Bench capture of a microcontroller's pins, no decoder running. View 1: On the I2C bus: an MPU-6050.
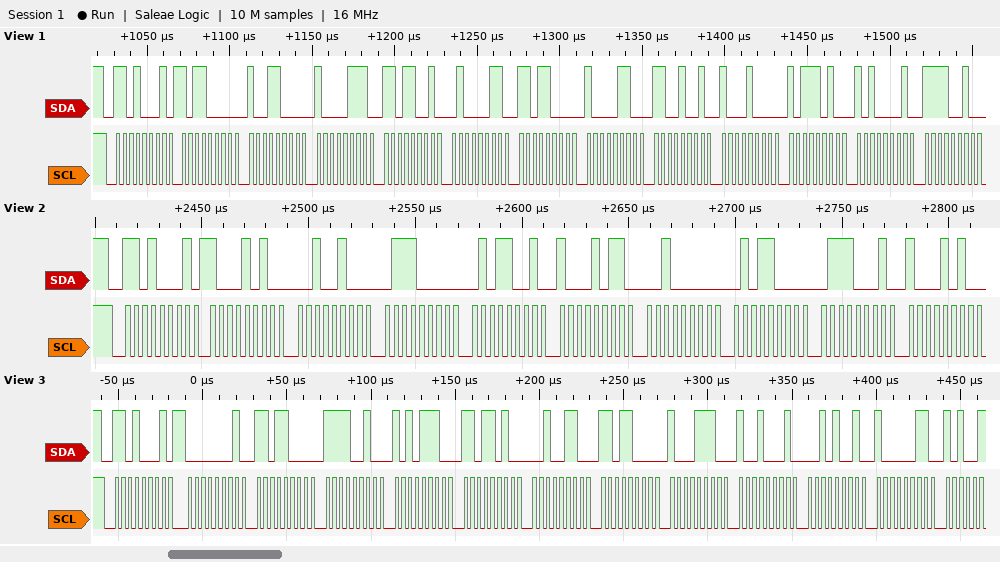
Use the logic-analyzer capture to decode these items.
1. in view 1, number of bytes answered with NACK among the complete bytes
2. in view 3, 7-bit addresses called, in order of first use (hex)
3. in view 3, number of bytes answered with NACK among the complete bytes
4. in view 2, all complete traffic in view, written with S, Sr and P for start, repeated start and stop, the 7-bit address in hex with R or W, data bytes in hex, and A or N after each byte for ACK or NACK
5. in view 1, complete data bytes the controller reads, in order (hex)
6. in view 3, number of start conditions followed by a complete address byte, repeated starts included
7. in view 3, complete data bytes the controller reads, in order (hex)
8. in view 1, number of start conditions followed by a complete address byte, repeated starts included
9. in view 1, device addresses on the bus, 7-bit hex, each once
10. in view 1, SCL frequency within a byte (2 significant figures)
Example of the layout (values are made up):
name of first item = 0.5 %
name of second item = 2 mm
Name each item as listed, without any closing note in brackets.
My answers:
in view 1, number of bytes answered with NACK among the complete bytes = 0
in view 3, 7-bit addresses called, in order of first use = 0x68
in view 3, number of bytes answered with NACK among the complete bytes = 0
in view 2, all complete traffic in view, written with S, Sr and P for start, repeated start and stop, the 7-bit address in hex with R or W, data bytes in hex, and A or N after each byte for ACK or NACK = S 68R A 8A A 24 A 70 A 59 A 8B A 20 A 58 A 71 A 8A A
in view 1, complete data bytes the controller reads, in order = B0 98 87 D9 43 D8 86 C9 88 BA A1 F2
in view 3, number of start conditions followed by a complete address byte, repeated starts included = 1
in view 3, complete data bytes the controller reads, in order = 01 D8 F2 AE DA 26 D8 8E 91 29 83
in view 1, number of start conditions followed by a complete address byte, repeated starts included = 1
in view 1, device addresses on the bus, 7-bit hex, each once = 0x68
in view 1, SCL frequency within a byte = 250 kHz
